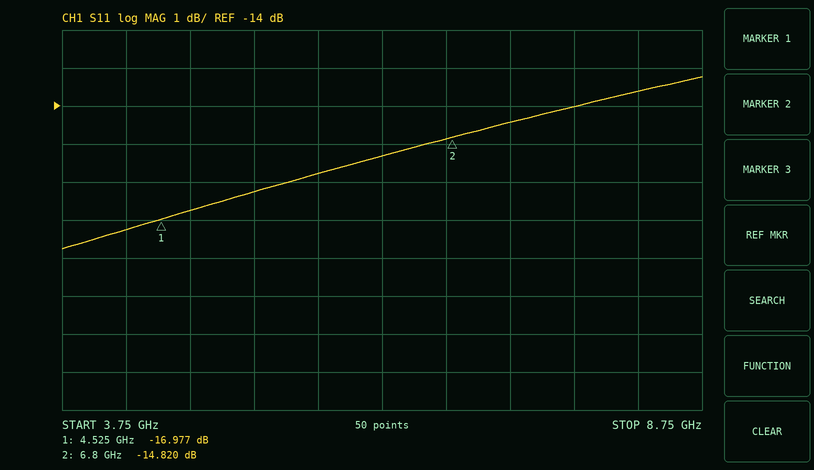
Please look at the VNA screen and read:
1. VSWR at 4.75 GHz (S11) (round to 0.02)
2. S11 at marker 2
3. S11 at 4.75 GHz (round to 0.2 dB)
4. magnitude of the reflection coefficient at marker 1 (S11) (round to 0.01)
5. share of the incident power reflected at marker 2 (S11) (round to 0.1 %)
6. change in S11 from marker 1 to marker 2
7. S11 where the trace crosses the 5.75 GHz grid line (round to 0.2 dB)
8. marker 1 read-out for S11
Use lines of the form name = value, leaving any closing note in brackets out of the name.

VSWR at 4.75 GHz (S11) = 1.34
S11 at marker 2 = -14.820 dB
S11 at 4.75 GHz = -16.8 dB
magnitude of the reflection coefficient at marker 1 (S11) = 0.14
share of the incident power reflected at marker 2 (S11) = 3.3 %
change in S11 from marker 1 to marker 2 = 2.157 dB
S11 where the trace crosses the 5.75 GHz grid line = -15.8 dB
marker 1 read-out for S11 = -16.977 dB
